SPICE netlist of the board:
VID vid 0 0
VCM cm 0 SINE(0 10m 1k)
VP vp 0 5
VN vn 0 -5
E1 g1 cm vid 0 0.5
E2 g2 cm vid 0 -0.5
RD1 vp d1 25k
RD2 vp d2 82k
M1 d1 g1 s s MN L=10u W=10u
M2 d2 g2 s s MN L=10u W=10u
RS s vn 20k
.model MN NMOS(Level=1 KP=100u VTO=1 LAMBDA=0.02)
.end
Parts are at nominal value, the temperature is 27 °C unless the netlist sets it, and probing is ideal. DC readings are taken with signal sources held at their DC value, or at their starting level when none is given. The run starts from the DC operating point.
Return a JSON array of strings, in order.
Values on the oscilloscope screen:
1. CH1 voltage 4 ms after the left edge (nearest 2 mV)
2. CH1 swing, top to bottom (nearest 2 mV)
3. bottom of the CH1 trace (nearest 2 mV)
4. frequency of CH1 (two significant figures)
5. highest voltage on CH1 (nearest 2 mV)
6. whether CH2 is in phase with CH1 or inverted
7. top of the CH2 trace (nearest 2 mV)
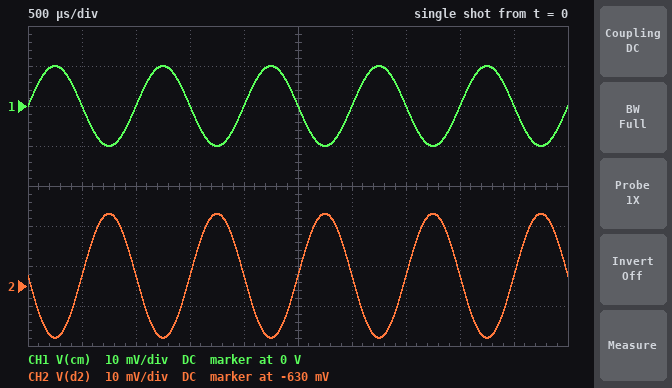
["0 V", "20 mV", "-10 mV", "1.0 kHz", "10 mV", "inverted", "-612 mV"]
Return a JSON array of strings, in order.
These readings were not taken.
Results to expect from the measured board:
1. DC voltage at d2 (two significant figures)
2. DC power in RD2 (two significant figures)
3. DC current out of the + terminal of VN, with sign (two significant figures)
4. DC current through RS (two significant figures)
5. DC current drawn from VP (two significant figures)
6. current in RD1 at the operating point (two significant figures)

["-630 mV", "390 µW", "-140 µA", "140 µA", "140 µA", "74 µA"]
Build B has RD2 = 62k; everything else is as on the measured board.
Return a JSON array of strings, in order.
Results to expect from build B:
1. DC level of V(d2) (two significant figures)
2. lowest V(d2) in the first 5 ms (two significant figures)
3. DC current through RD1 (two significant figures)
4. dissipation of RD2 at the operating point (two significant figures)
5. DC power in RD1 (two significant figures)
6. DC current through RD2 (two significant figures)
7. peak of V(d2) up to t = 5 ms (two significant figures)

["680 mV", "670 mV", "73 µA", "300 µW", "130 µW", "70 µA", "690 mV"]
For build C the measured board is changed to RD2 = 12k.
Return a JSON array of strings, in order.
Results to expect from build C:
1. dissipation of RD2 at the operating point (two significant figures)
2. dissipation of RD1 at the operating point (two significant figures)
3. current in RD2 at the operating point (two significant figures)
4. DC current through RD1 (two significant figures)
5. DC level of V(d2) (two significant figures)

["63 µW", "130 µW", "72 µA", "71 µA", "4.1 V"]
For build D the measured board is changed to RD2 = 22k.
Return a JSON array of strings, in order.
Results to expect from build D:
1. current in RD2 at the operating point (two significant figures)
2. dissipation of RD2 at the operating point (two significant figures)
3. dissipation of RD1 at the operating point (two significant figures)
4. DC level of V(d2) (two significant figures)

["72 µA", "110 µW", "130 µW", "3.4 V"]
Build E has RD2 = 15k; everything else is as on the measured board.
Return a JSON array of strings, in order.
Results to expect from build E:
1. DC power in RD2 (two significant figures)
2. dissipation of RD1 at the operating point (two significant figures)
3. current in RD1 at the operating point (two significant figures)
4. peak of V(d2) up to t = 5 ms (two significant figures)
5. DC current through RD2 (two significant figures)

["78 µW", "130 µW", "71 µA", "3.9 V", "72 µA"]
